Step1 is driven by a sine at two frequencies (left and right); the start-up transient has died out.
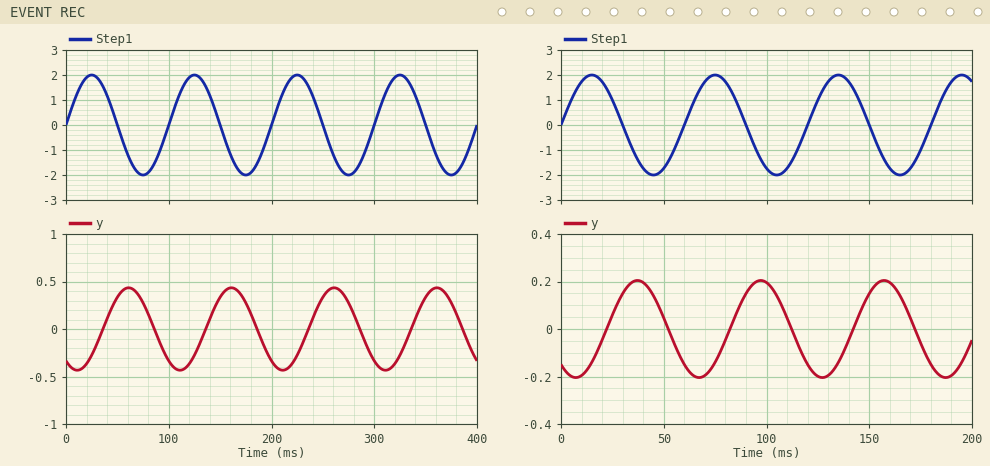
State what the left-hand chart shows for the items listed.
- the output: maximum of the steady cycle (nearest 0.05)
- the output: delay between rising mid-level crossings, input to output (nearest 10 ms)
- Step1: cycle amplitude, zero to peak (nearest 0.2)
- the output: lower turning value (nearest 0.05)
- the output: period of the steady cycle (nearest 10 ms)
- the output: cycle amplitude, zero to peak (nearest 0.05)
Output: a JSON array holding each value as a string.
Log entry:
["0.45", "40 ms", "2.0", "-0.45", "100 ms", "0.45"]
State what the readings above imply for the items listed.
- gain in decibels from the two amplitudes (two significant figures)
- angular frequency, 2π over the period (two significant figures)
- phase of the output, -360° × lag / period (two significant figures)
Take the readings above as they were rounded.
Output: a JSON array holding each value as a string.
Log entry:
["-13 dB", "0.063 rad/ms", "-140°"]
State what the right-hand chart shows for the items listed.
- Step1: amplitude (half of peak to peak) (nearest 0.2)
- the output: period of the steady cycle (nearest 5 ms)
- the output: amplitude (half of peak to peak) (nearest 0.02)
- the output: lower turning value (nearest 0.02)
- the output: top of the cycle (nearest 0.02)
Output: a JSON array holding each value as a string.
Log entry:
["2.0", "60 ms", "0.20", "-0.20", "0.20"]
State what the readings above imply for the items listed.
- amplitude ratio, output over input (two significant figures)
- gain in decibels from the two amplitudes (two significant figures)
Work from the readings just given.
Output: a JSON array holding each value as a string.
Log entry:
["0.10", "-20 dB"]
